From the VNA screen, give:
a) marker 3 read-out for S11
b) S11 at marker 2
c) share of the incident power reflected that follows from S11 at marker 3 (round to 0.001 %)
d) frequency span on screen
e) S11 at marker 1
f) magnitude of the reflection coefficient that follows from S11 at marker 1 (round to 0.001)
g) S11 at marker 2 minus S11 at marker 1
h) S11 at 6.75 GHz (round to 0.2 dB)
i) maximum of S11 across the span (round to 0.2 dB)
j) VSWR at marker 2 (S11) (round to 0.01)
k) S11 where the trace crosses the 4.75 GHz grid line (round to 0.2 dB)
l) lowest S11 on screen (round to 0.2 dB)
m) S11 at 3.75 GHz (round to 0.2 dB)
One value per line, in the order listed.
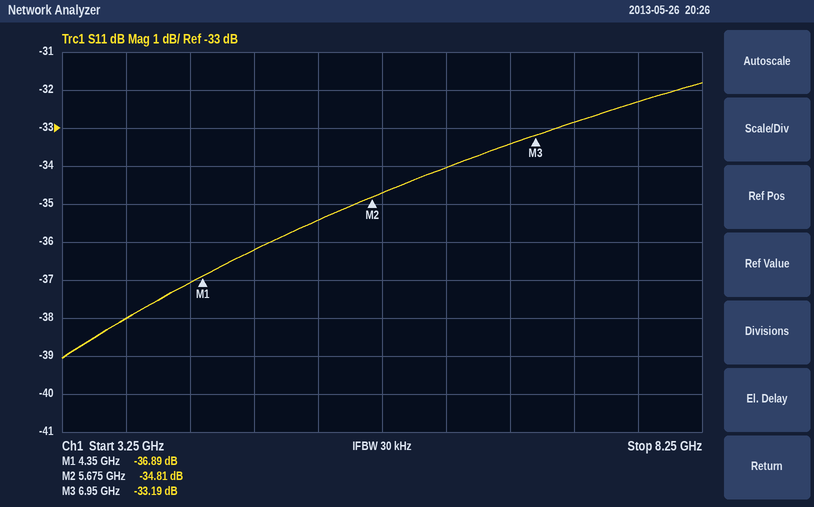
-33.19 dB
-34.81 dB
0.048 %
5 GHz
-36.89 dB
0.014
2.08 dB
-33.4 dB
-31.8 dB
1.04
-36.2 dB
-39.0 dB
-38.0 dB
